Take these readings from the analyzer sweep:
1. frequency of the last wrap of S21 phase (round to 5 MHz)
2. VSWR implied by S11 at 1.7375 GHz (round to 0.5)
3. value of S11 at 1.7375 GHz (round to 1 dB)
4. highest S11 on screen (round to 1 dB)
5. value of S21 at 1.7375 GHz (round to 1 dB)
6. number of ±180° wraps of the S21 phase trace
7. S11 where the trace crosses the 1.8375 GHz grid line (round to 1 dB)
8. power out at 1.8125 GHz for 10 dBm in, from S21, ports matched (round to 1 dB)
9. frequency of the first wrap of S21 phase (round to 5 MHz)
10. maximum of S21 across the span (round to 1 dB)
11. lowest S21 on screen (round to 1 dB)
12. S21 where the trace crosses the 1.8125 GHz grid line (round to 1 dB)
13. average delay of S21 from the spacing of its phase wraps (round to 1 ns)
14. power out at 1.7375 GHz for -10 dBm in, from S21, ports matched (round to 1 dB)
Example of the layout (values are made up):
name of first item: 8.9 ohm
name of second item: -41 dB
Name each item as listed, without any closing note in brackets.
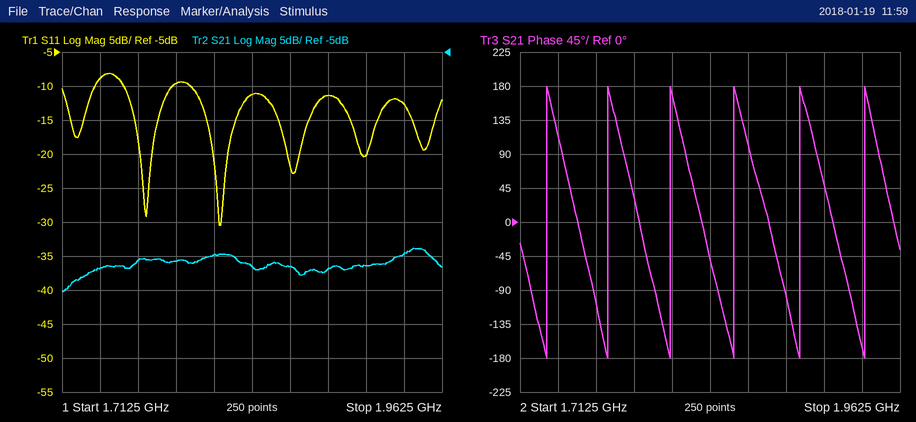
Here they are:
frequency of the last wrap of S21 phase: 1.940 GHz
VSWR implied by S11 at 1.7375 GHz: 2.0
value of S11 at 1.7375 GHz: -9 dB
highest S11 on screen: -8 dB
value of S21 at 1.7375 GHz: -37 dB
number of ±180° wraps of the S21 phase trace: 6
S11 where the trace crosses the 1.8375 GHz grid line: -11 dB
power out at 1.8125 GHz for 10 dBm in, from S21, ports matched: -25 dBm
frequency of the first wrap of S21 phase: 1.730 GHz
maximum of S21 across the span: -34 dB
lowest S21 on screen: -40 dB
S21 where the trace crosses the 1.8125 GHz grid line: -35 dB
average delay of S21 from the spacing of its phase wraps: 24 ns
power out at 1.7375 GHz for -10 dBm in, from S21, ports matched: -47 dBm
